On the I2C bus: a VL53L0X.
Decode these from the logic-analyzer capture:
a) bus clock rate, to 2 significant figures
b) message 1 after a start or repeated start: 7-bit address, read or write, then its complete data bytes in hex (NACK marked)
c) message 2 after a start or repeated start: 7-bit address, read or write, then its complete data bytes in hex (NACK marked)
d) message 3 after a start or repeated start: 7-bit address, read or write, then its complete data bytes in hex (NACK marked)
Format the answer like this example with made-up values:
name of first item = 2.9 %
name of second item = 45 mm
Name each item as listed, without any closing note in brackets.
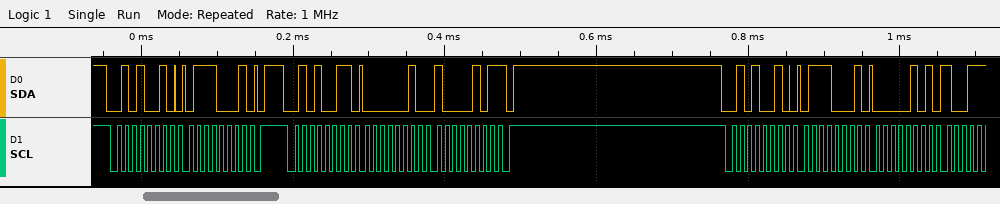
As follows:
bus clock rate, to 2 significant figures = 100 kHz
message 1 after a start or repeated start: 7-bit address, read or write, then its complete data bytes in hex = 0x29 write: 71
message 2 after a start or repeated start: 7-bit address, read or write, then its complete data bytes in hex = 0x29 read: 02 85 NACK
message 3 after a start or repeated start: 7-bit address, read or write, then its complete data bytes in hex = 0x29 write: 71 05
